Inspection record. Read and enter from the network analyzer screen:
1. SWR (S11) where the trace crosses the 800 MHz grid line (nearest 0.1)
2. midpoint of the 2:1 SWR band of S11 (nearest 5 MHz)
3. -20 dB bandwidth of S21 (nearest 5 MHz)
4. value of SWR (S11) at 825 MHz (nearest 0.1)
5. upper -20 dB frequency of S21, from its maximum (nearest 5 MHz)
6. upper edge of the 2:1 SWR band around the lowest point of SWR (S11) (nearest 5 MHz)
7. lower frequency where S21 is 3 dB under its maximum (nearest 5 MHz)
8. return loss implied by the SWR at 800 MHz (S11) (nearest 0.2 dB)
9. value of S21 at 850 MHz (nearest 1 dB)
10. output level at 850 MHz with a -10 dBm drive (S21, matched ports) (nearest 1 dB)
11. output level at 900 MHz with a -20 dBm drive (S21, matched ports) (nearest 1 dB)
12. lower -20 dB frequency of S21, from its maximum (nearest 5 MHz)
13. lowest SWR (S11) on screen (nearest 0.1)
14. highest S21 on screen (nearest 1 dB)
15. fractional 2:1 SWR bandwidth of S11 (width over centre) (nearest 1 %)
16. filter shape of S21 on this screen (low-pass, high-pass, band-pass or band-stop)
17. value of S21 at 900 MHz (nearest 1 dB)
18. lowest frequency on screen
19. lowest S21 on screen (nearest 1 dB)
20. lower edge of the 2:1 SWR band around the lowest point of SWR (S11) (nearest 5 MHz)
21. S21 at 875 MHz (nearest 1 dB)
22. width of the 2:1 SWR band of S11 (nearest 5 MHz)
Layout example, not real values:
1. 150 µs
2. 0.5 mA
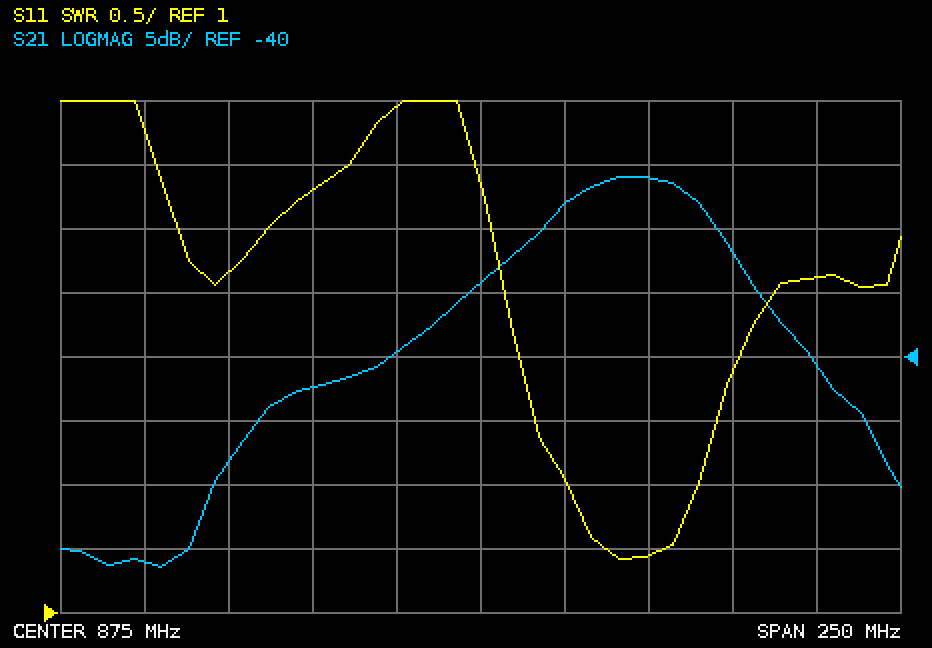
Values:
1. 3.7
2. 920 MHz
3. 185 MHz
4. 4.3
5. 990 MHz
6. 940 MHz
7. 895 MHz
8. 4.8 dB
9. -40 dB
10. -50 dBm
11. -48 dBm
12. 805 MHz
13. 1.4
14. -26 dB
15. 4 %
16. band-pass
17. -28 dB
18. 750 MHz
19. -56 dB
20. 900 MHz
21. -34 dB
22. 40 MHz
